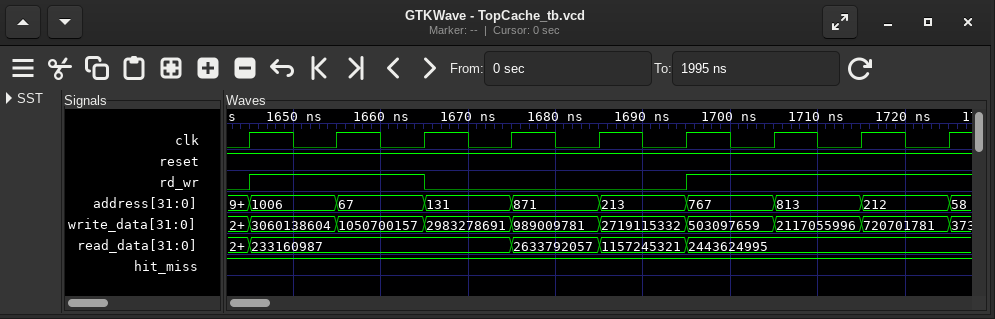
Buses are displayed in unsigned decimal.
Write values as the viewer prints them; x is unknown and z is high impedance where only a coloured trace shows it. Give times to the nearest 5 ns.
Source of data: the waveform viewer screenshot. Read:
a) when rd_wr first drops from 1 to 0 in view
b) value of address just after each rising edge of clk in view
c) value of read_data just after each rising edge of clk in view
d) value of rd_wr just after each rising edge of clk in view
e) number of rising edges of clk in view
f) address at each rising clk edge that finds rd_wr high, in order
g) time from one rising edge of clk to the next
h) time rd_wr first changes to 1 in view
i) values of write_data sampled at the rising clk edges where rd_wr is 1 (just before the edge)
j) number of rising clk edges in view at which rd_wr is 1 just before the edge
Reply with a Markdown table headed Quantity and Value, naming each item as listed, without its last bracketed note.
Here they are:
| Quantity | Value |
|---|---|
| when rd_wr first drops from 1 to 0 in view | 1665 ns |
| value of address just after each rising edge of clk in view | 1006, 67, 131, 871, 213, 767, 813, 212, 58 |
| value of read_data just after each rising edge of clk in view | 233160987, 233160987, 233160987, 2633792057, 1157245321, 2443624995, 2443624995, 2443624995, 2443624995 |
| value of rd_wr just after each rising edge of clk in view | 1 1 0 0 0 1 1 1 1 |
| number of rising edges of clk in view | 9 |
| address at each rising clk edge that finds rd_wr high, in order | 1006, 67, 767, 813, 212 |
| time from one rising edge of clk to the next | 10 ns |
| time rd_wr first changes to 1 in view | 1645 ns |
| values of write_data sampled at the rising clk edges where rd_wr is 1 | 3060138604, 1050700157, 503097659, 2117055996, 720701781 |
| number of rising clk edges in view at which rd_wr is 1 just before the edge | 5 |
